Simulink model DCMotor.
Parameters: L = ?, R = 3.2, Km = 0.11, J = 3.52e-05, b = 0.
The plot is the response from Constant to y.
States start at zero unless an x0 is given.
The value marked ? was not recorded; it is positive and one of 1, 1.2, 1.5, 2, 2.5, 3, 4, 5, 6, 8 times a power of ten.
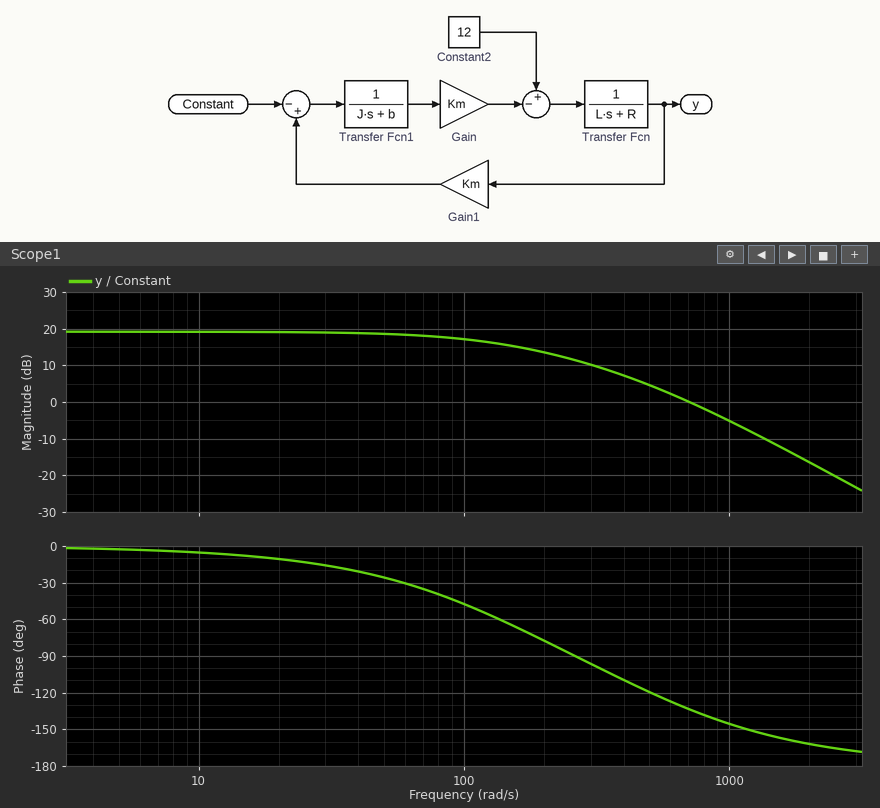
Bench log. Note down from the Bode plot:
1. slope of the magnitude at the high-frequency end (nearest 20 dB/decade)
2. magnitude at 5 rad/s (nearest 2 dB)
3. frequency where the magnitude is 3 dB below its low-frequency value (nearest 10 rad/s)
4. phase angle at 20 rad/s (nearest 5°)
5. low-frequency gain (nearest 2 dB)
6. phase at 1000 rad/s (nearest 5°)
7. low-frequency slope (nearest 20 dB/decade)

-40 dB/decade
20 dB
130 rad/s
-10°
20 dB
-145°
0 dB/decade
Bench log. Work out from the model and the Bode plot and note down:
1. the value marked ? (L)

0.005
